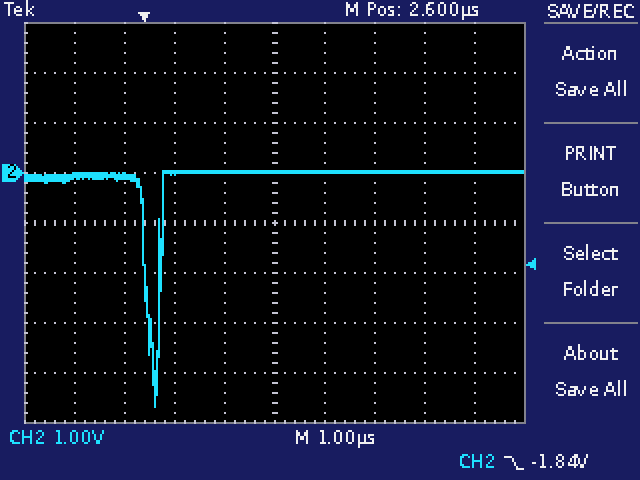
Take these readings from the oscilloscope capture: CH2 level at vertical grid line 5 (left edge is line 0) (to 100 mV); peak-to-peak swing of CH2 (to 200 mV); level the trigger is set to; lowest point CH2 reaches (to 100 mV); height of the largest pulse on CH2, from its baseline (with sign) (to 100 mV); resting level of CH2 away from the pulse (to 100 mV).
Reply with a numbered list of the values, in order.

1. 0.0 V
2. 4.8 V
3. -1.84 V
4. -4.7 V
5. -4.7 V
6. 0.0 V
